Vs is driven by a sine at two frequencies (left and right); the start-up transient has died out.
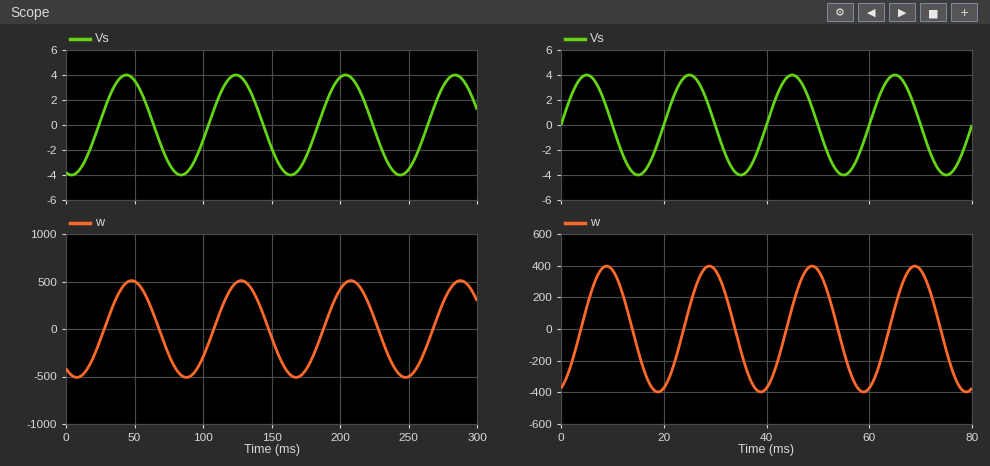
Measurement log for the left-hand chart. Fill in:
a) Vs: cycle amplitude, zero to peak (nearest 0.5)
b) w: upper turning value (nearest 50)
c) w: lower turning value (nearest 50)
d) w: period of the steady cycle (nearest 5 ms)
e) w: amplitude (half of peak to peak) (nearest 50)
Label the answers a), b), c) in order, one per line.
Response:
a) 4.0
b) 500
c) -500
d) 80 ms
e) 500
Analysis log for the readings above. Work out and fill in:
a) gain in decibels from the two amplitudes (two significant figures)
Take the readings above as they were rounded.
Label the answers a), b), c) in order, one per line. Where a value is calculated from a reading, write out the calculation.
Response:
a) 20 log10(500 / 4) = 42 dB
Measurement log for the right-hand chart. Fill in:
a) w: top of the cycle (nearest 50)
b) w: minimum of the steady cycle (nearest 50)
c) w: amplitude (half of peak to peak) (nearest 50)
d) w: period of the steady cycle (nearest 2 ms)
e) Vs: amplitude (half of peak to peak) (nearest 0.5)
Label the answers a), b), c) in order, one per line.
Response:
a) 400
b) -400
c) 400
d) 20 ms
e) 4.0
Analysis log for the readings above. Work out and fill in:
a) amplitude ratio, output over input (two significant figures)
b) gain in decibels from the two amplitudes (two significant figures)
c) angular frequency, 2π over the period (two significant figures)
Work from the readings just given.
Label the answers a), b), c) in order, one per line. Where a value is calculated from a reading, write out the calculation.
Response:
a) 400 / 4 = 100
b) 20 log10(400 / 4) = 40 dB
c) 2π / 20 = 0.31 rad/ms
